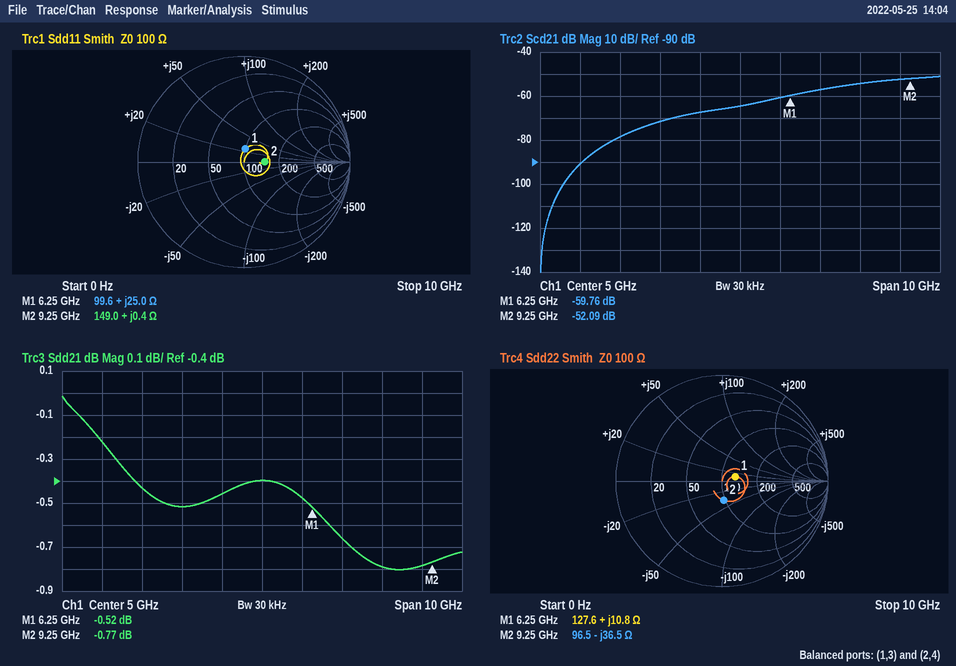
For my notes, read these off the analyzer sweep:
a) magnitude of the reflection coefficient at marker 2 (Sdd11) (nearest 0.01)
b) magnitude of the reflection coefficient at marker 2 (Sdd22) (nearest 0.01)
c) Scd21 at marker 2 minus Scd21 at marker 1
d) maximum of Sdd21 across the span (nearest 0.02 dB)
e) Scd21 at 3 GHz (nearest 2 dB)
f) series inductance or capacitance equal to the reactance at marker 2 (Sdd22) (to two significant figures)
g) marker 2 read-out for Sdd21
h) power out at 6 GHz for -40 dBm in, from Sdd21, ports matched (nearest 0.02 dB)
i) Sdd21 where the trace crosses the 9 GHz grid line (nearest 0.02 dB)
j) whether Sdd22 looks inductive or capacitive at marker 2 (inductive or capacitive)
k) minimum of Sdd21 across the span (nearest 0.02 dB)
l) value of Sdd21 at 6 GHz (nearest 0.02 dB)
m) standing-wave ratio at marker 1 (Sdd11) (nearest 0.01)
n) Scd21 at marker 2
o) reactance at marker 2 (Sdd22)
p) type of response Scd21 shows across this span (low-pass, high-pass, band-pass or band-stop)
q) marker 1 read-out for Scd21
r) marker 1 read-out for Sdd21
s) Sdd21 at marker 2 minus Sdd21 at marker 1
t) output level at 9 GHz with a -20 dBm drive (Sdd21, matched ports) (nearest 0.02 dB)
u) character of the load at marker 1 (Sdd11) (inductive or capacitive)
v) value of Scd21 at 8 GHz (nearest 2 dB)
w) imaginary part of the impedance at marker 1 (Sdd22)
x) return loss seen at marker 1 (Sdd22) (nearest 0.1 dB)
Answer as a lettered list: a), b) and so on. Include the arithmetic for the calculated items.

a) 0.20
b) 0.18
c) -52.09 − (-59.76) = 7.67 dB
d) -0.02 dB
e) -72 dB
f) C = 1/(2π × 9.25 GHz × 36.5 Ω) ≈ 471 fF, so 470 fF to two significant figures
g) -0.77 dB
h) -40 dBm + (-0.48 dB) = -40.48 dBm
i) -0.78 dB
j) capacitive
k) -0.80 dB
l) -0.48 dB
m) 1.28
n) -52.09 dB
o) -36.5 Ω
p) high-pass
q) -59.76 dB
r) -0.52 dB
s) -0.77 − (-0.52) = -0.25 dB
t) -20 dBm + (-0.78 dB) = -20.78 dBm
u) inductive
v) -54 dB
w) +10.8 Ω
x) 17.7 dB
